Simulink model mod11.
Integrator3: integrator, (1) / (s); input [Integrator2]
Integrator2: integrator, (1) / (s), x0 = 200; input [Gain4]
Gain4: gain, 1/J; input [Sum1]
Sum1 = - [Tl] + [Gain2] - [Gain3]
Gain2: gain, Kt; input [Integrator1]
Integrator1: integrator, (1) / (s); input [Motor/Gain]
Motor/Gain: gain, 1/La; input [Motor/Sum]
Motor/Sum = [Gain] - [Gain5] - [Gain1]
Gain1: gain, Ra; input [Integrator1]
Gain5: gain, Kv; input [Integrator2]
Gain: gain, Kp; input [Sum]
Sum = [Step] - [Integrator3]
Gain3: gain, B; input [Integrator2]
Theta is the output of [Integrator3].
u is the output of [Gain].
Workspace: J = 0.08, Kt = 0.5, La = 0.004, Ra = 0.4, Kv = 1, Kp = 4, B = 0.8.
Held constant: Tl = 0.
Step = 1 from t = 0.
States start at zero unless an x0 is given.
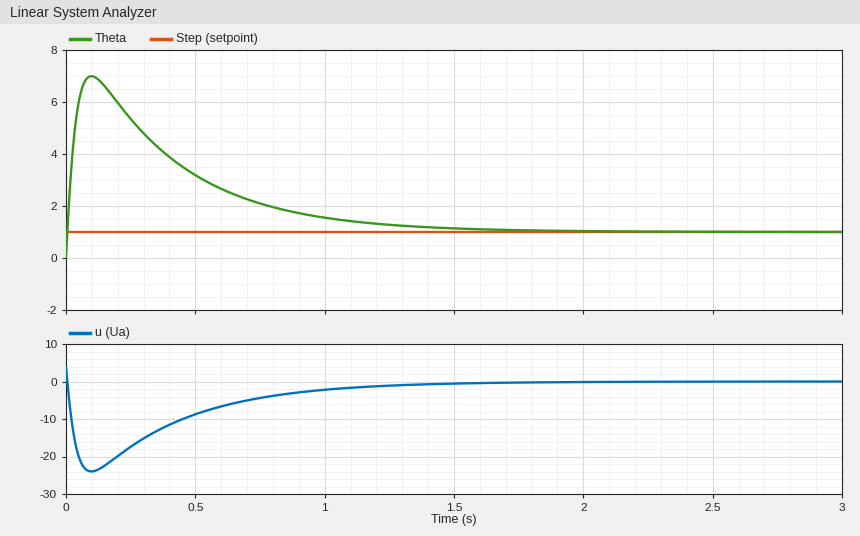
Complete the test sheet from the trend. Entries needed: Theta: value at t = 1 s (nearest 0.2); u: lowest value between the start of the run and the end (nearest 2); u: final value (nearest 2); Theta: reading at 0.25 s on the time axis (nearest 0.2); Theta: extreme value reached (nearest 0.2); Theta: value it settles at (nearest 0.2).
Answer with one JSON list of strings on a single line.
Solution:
["1.6", "-24", "0", "5.4", "7.0", "1.0"]
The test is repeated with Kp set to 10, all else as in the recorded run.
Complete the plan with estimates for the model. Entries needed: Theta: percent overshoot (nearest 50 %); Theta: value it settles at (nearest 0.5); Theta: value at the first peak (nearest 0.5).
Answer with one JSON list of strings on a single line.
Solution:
["550 %", "1.0", "6.5"]
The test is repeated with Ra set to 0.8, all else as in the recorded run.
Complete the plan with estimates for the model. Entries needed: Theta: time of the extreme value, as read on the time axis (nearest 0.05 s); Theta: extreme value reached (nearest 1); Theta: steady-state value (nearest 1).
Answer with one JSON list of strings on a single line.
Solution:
["0.15 s", "10", "1"]
